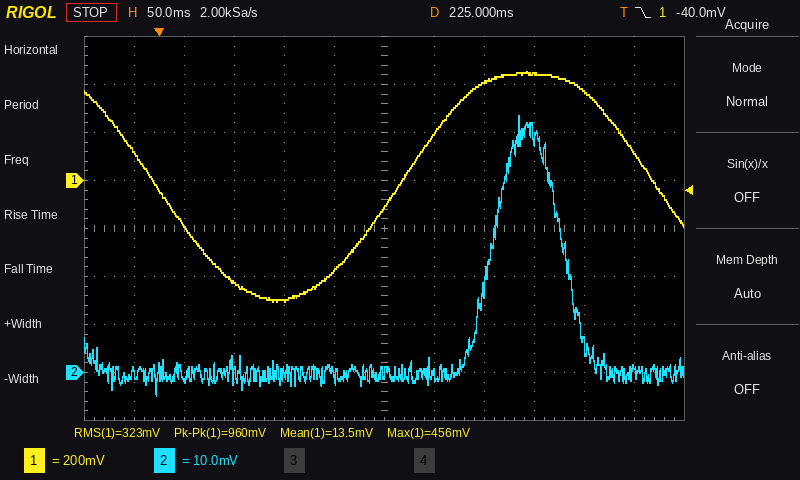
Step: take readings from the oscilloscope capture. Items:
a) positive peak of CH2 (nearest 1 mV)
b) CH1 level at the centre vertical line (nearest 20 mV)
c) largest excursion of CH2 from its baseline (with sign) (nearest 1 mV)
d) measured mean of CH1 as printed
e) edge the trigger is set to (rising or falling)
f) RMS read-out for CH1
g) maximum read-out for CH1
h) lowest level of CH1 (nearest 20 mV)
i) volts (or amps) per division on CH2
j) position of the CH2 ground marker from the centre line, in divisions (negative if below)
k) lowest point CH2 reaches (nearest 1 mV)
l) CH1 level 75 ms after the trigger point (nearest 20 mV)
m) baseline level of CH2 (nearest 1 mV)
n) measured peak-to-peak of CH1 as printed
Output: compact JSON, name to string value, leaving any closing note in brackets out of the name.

{"positive peak of CH2": "54 mV", "CH1 level at the centre vertical line": "-120 mV", "largest excursion of CH2 from its baseline (with sign)": "+54 mV", "measured mean of CH1 as printed": "13.5 mV", "edge the trigger is set to": "falling", "RMS read-out for CH1": "323 mV", "maximum read-out for CH1": "456 mV", "lowest level of CH1": "-500 mV", "volts (or amps) per division on CH2": "10 mV", "position of the CH2 ground marker from the centre line, in divisions": "-3.0 div", "lowest point CH2 reaches": "-5 mV", "CH1 level 75 ms after the trigger point": "-420 mV", "baseline level of CH2": "0 mV", "measured peak-to-peak of CH1 as printed": "960 mV"}
